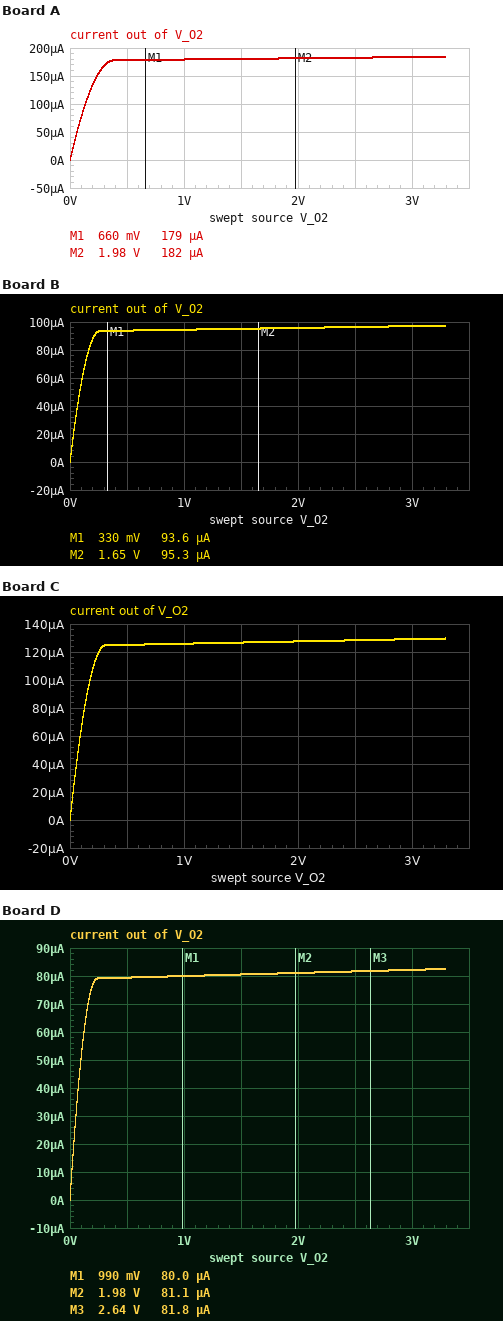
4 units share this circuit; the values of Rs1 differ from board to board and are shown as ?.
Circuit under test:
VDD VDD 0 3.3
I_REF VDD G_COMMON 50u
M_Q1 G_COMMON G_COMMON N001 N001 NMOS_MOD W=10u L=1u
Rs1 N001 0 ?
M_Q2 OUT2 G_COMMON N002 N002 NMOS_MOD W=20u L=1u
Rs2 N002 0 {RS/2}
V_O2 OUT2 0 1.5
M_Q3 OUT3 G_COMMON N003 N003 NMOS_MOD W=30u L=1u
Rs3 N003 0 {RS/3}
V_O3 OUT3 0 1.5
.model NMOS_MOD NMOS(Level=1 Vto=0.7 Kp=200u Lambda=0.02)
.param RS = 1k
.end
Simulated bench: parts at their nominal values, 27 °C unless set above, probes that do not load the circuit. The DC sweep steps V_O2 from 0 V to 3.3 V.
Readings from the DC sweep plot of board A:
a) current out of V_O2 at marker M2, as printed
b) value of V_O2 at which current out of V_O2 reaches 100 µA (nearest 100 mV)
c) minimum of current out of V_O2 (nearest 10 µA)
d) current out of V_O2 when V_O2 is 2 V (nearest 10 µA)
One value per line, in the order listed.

182 µA
100 mV
0 A
180 µA
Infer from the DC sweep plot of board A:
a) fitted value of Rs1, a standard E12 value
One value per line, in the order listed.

3.3 kΩ
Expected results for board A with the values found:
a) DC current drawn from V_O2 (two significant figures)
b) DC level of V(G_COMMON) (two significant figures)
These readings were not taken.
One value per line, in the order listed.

180 µA
1.1 V
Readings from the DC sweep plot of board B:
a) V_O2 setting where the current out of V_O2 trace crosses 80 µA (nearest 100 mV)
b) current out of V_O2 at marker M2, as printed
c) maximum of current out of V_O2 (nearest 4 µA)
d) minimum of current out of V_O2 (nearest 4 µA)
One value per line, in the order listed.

200 mV
95.3 µA
96 µA
0 A
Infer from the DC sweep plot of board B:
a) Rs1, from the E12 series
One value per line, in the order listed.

820 Ω
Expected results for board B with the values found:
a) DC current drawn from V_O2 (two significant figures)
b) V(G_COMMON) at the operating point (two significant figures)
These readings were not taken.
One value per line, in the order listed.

95 µA
960 mV
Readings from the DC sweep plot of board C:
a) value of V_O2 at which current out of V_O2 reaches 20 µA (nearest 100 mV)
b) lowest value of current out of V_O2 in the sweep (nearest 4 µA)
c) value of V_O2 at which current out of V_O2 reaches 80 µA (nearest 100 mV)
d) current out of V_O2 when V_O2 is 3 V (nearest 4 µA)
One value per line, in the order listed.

0 V
0 A
100 mV
128 µA
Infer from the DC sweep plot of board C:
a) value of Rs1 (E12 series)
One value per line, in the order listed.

1.8 kΩ
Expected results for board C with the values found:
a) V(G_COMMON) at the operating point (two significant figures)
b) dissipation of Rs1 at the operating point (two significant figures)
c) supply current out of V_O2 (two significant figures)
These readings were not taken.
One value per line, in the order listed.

1.0 V
4.5 µW
130 µA
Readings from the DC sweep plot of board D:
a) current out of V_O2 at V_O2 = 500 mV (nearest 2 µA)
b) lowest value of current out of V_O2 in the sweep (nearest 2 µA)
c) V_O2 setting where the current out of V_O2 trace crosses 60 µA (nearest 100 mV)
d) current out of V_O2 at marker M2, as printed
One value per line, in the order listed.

80 µA
0 A
100 mV
81.1 µA
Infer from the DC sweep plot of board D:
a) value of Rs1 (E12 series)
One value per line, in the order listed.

330 Ω
